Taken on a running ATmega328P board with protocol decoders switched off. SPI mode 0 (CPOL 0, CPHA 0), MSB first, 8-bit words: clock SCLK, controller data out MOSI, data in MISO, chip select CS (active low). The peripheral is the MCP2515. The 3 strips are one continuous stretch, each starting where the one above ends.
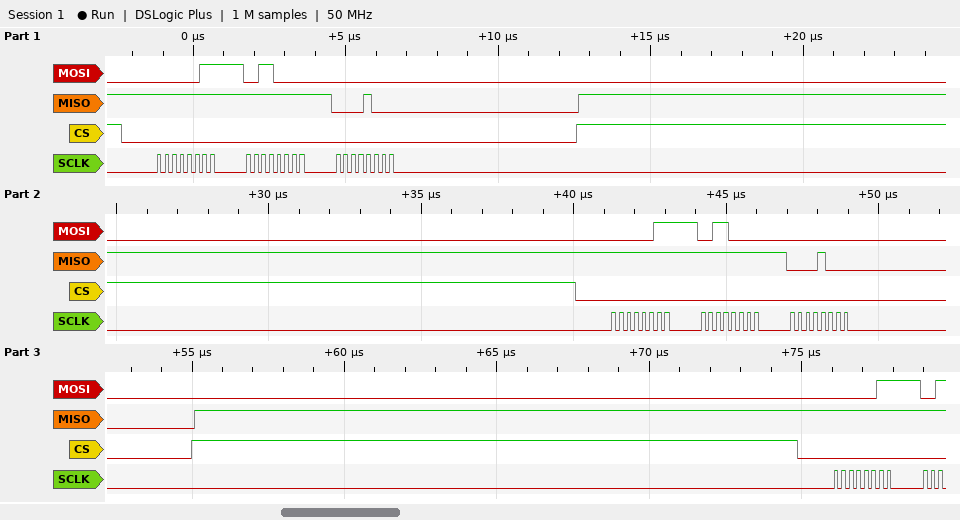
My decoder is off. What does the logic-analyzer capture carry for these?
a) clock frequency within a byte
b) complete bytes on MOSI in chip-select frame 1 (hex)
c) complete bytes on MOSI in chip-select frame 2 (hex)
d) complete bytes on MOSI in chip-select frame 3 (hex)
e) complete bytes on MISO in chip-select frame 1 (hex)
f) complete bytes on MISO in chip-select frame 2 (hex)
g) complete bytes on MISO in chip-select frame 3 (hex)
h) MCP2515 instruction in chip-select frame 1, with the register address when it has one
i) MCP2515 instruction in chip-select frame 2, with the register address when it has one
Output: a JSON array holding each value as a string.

["4 MHz", "03 30 00", "03 30 00", "03", "FF FF 08", "FF FF 08", "FF", "READ 0x30", "READ 0x30"]
